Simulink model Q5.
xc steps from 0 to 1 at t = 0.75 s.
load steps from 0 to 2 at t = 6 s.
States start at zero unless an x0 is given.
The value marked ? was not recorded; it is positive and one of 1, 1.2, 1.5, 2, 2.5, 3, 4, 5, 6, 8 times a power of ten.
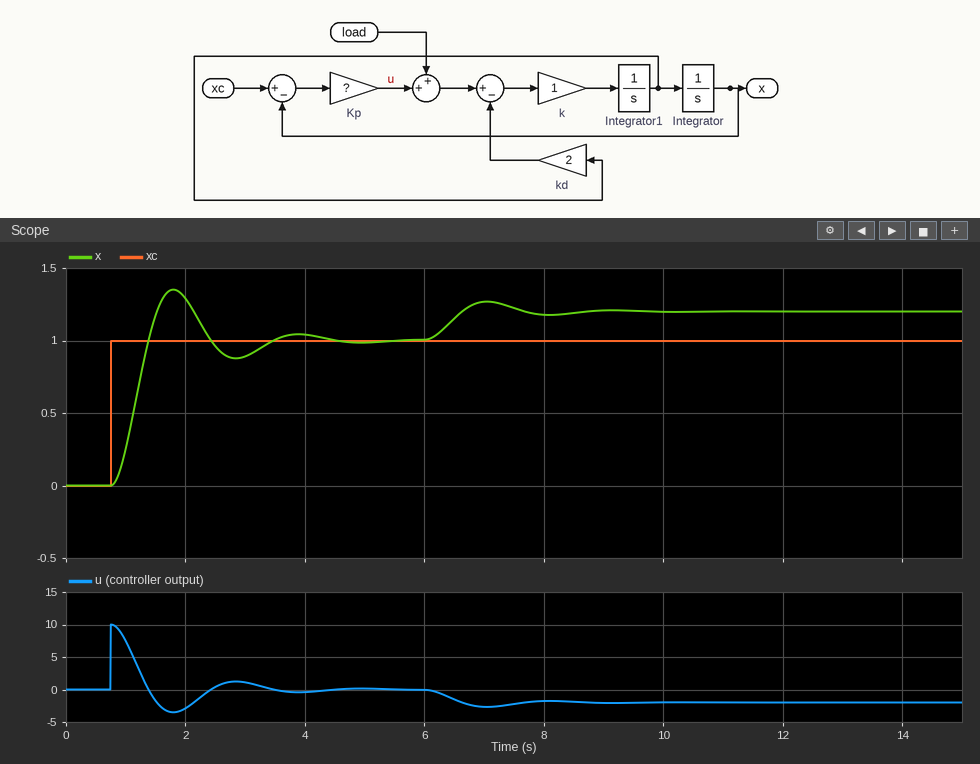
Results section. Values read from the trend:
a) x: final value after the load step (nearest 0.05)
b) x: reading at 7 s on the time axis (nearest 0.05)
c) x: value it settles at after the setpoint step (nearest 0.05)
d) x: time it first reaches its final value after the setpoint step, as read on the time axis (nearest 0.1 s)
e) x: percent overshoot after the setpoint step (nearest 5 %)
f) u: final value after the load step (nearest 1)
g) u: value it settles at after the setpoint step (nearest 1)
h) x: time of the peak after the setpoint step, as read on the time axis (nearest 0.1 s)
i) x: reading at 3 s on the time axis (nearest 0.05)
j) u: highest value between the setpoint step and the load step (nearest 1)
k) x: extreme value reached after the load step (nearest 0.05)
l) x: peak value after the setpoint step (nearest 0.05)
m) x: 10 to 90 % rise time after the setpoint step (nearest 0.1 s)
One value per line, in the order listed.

1.20
1.25
1.00
1.4 s
35 %
-2
0
1.8 s
0.90
10
1.25
1.35
0.4 s
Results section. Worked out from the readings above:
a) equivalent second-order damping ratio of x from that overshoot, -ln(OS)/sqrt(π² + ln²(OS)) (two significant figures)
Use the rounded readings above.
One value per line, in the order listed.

0.32
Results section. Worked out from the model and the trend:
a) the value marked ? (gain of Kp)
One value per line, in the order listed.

10
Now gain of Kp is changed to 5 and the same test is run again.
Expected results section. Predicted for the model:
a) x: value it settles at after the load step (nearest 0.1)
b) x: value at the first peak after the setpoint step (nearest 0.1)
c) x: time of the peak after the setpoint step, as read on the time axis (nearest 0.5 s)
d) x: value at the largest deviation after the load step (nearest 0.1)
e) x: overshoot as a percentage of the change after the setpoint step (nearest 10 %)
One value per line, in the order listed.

1.4
1.2
2.5 s
1.5
20 %
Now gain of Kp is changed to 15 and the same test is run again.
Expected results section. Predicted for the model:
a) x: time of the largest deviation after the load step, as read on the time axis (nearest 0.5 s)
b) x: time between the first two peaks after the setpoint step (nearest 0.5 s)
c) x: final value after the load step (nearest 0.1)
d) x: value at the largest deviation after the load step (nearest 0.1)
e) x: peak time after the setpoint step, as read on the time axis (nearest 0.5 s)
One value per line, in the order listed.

7.0 s
1.5 s
1.1
1.2
1.5 s
